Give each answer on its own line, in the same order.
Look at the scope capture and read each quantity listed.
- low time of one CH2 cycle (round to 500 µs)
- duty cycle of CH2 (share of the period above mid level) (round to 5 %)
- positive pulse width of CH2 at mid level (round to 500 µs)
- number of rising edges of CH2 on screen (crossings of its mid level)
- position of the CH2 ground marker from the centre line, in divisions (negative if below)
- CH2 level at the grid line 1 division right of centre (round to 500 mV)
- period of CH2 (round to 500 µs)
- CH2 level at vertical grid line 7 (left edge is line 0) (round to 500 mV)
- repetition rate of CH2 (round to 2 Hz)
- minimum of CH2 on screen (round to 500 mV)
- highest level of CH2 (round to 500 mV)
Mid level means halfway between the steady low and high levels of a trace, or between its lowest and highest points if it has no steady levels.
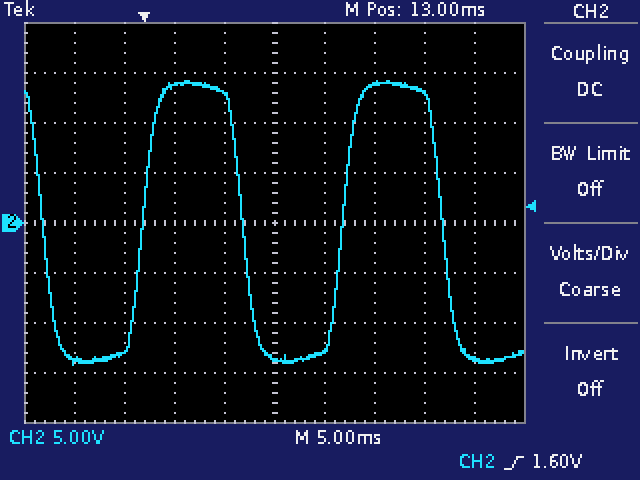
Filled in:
10.0 ms
50 %
10.0 ms
2
0.0 div
-12.5 V
20.0 ms
14.0 V
50 Hz
-14.0 V
14.0 V
